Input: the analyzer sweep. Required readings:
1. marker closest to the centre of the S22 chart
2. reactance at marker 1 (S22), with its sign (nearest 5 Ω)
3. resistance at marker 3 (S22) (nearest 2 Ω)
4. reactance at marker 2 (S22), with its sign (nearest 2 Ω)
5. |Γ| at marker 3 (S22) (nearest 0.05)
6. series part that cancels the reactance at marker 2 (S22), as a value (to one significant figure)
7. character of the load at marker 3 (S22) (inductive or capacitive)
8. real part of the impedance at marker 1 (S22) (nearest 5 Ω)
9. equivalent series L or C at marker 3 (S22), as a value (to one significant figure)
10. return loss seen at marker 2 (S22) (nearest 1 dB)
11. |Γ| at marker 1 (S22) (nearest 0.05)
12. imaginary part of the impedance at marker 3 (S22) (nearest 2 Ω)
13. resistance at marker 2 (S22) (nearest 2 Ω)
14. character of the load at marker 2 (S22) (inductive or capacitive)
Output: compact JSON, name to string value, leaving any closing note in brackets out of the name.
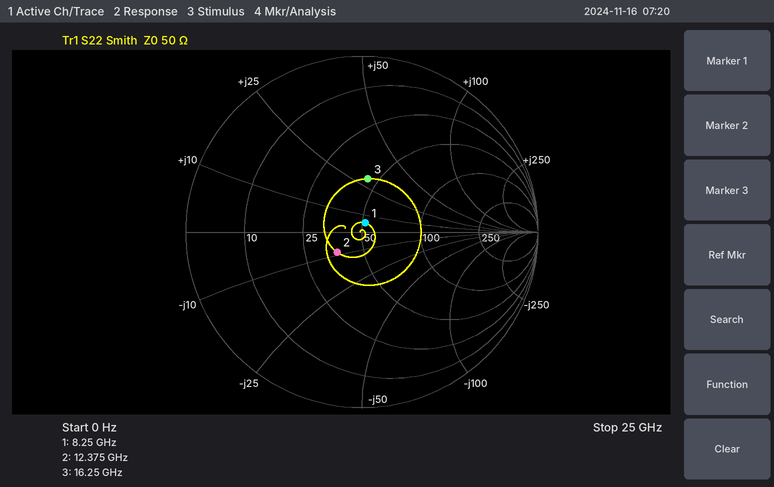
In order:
{"marker closest to the centre of the S22 chart": "marker 1", "reactance at marker 1 (S22), with its sign": "+5 Ω", "resistance at marker 3 (S22)": "44 Ω", "reactance at marker 2 (S22), with its sign": "-8 Ω", "|Γ| at marker 3 (S22)": "0.30", "series part that cancels the reactance at marker 2 (S22), as a value": "100 pH", "character of the load at marker 3 (S22)": "inductive", "real part of the impedance at marker 1 (S22)": "50 Ω", "equivalent series L or C at marker 3 (S22), as a value": "300 pH", "return loss seen at marker 2 (S22)": "15 dB", "|Γ| at marker 1 (S22)": "0.05", "imaginary part of the impedance at marker 3 (S22)": "+30 Ω", "resistance at marker 2 (S22)": "36 Ω", "character of the load at marker 2 (S22)": "capacitive"}
